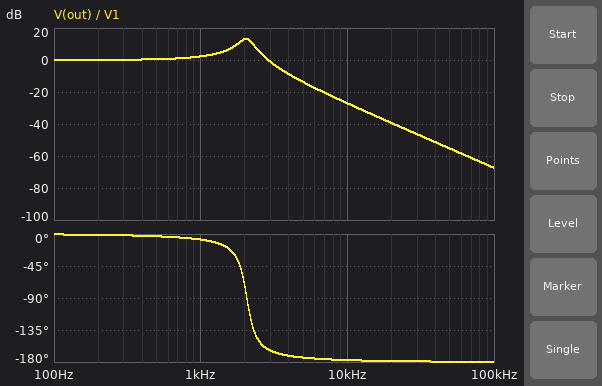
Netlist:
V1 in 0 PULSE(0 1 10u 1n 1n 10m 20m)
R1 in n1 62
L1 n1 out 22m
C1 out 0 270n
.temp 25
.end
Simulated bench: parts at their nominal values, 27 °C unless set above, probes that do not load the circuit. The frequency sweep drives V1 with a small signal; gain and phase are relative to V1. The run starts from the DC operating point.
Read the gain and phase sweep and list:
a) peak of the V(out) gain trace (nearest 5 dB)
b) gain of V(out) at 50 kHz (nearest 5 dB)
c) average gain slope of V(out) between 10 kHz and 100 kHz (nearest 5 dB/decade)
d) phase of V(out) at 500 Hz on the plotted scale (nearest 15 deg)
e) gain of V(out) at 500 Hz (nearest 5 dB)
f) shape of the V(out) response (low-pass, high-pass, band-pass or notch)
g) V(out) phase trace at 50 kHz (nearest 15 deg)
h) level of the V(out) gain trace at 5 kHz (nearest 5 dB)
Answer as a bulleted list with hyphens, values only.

- 15 dB
- -55 dB
- -40 dB/decade
- 0 deg
- 0 dB
- low-pass
- -180 deg
- -15 dB
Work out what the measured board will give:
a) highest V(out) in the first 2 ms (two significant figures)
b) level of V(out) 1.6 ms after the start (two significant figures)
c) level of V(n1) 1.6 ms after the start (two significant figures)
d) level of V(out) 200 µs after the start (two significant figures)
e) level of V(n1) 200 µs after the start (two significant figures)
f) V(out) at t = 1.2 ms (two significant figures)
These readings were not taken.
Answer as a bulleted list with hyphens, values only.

- 1.7 V
- 1.0 V
- 980 mV
- 1.5 V
- 890 mV
- 1.2 V
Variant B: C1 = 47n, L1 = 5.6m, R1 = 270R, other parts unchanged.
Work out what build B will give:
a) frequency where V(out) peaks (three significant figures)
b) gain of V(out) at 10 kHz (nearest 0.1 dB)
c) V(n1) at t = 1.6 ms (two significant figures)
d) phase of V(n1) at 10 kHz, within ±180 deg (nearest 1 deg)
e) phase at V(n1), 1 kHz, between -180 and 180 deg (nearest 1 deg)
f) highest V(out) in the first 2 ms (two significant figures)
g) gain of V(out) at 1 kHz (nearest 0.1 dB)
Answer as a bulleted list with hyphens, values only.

- 8.17 kHz
- 2.0 dB
- 1.0 V
- 87 deg
- -5 deg
- 1.3 V
- 0.1 dB
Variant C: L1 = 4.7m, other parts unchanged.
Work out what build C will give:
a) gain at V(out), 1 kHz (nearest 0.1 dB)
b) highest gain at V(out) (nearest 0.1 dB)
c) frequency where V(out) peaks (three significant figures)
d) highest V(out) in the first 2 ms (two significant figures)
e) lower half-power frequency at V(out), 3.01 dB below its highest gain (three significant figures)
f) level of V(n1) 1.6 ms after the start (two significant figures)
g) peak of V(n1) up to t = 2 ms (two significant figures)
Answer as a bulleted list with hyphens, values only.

- 0.4 dB
- 6.8 dB
- 4.21 kHz
- 1.5 V
- 2.94 kHz
- 1.0 V
- 1.2 V
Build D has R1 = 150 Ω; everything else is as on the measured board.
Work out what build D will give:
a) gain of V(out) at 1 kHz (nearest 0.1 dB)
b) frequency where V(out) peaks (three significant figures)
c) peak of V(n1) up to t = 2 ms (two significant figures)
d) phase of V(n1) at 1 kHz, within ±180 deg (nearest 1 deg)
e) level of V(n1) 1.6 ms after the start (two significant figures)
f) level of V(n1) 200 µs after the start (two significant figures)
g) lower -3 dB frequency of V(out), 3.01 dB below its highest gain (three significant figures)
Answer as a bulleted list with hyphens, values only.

- 1.9 dB
- 1.92 kHz
- 1.2 V
- -18 deg
- 1.0 V
- 800 mV
- 1.23 kHz
